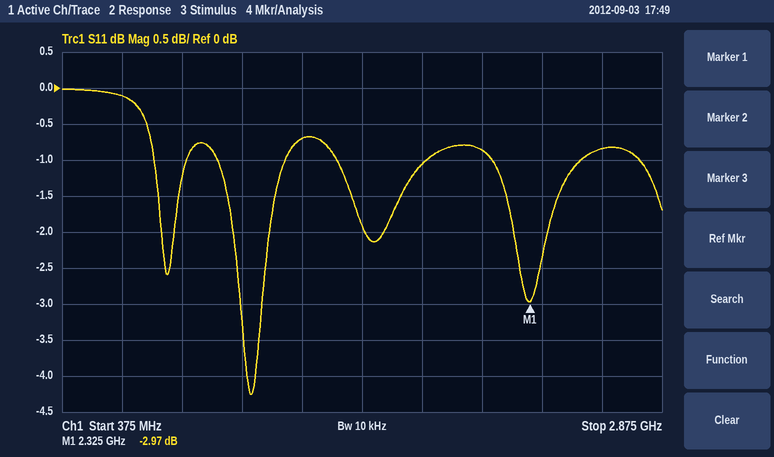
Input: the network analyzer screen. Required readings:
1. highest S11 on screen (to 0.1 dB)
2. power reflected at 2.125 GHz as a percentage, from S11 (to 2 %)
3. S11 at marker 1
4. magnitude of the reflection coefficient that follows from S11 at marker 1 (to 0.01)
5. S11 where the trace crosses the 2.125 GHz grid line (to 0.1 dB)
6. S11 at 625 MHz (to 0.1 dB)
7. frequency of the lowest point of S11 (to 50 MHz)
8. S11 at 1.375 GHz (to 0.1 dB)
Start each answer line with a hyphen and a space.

- 0.0 dB
- 82 %
- -2.97 dB
- 0.71
- -0.9 dB
- -0.1 dB
- 1.15 GHz
- -0.7 dB
